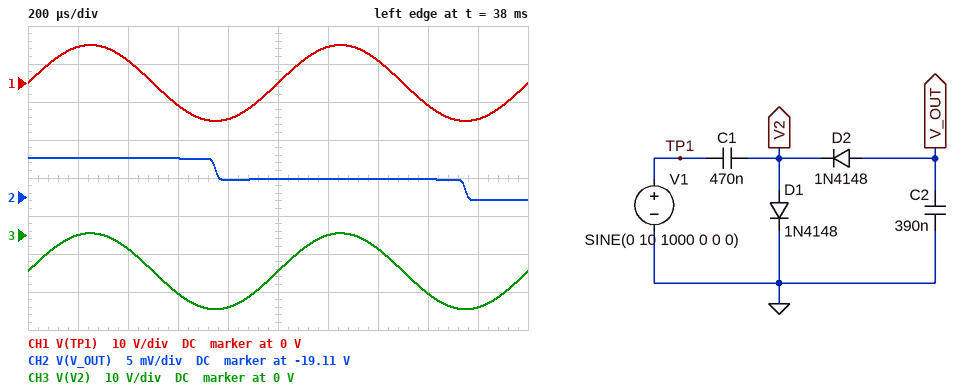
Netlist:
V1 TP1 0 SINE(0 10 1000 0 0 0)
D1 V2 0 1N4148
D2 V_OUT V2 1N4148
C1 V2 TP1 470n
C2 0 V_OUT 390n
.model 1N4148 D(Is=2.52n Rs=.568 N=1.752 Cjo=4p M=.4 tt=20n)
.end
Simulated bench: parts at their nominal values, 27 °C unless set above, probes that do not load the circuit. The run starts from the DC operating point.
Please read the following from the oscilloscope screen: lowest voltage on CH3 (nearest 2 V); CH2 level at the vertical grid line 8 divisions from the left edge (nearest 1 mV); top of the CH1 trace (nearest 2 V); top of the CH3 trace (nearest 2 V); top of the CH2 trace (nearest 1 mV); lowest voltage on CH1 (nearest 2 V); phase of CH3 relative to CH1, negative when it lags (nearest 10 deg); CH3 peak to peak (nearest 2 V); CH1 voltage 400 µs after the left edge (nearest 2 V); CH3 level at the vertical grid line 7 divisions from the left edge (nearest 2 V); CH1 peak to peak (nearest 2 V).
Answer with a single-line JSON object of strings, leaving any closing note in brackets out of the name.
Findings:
{"lowest voltage on CH3": "-20 V", "CH2 level at the vertical grid line 8 divisions from the left edge": "-19.103 V", "top of the CH1 trace": "10 V", "top of the CH3 trace": "0 V", "top of the CH2 trace": "-19.100 V", "lowest voltage on CH1": "-10 V", "phase of CH3 relative to CH1, negative when it lags": "0 deg", "CH3 peak to peak": "20 V", "CH1 voltage 400 µs after the left edge": "6 V", "CH3 level at the vertical grid line 7 divisions from the left edge": "-4 V", "CH1 peak to peak": "20 V"}
